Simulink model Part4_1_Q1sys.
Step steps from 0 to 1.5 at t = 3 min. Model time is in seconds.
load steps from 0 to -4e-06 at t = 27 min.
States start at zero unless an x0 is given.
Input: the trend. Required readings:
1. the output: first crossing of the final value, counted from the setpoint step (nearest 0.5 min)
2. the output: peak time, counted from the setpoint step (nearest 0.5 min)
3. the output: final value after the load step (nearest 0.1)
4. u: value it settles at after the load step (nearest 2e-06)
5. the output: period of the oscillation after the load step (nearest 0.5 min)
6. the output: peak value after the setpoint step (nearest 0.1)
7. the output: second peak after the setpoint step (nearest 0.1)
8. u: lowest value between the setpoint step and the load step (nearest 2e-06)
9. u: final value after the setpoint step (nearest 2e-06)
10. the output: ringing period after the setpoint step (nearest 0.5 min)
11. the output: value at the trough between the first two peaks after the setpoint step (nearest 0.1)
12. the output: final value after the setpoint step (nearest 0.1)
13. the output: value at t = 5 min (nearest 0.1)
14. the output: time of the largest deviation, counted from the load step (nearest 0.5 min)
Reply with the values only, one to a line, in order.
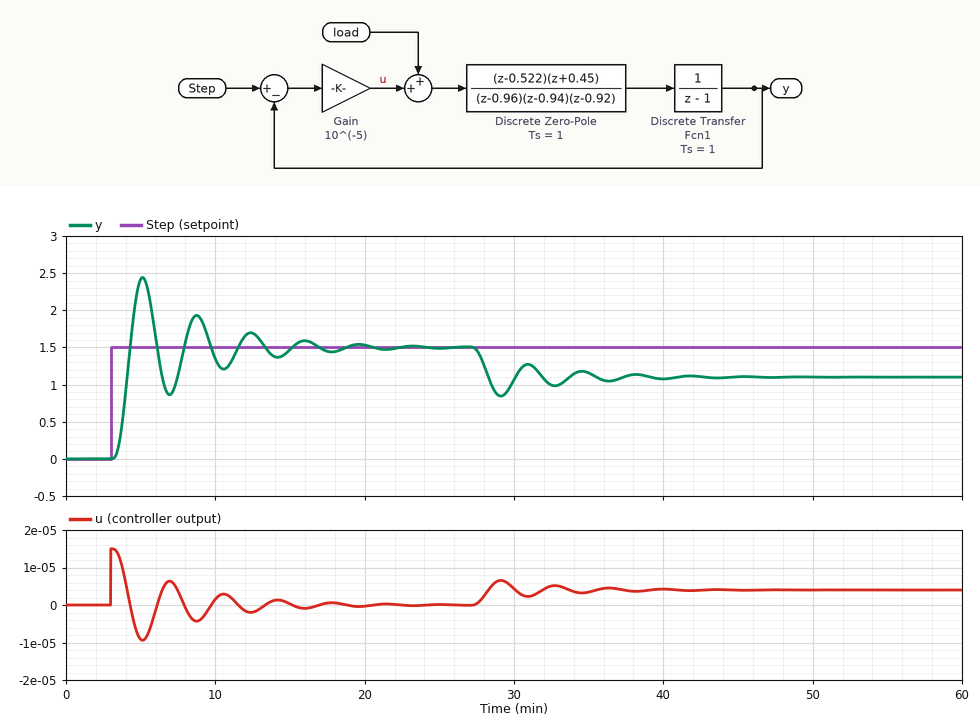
1.5 min
2.0 min
1.1
0.000004
3.5 min
2.4
1.9
-0.000010
0.000000
3.5 min
0.9
1.5
2.4
2.0 min
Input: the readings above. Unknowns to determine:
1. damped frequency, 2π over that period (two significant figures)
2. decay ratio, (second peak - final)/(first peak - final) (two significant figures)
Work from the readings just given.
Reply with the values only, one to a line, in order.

1.8 rad/min
0.44
